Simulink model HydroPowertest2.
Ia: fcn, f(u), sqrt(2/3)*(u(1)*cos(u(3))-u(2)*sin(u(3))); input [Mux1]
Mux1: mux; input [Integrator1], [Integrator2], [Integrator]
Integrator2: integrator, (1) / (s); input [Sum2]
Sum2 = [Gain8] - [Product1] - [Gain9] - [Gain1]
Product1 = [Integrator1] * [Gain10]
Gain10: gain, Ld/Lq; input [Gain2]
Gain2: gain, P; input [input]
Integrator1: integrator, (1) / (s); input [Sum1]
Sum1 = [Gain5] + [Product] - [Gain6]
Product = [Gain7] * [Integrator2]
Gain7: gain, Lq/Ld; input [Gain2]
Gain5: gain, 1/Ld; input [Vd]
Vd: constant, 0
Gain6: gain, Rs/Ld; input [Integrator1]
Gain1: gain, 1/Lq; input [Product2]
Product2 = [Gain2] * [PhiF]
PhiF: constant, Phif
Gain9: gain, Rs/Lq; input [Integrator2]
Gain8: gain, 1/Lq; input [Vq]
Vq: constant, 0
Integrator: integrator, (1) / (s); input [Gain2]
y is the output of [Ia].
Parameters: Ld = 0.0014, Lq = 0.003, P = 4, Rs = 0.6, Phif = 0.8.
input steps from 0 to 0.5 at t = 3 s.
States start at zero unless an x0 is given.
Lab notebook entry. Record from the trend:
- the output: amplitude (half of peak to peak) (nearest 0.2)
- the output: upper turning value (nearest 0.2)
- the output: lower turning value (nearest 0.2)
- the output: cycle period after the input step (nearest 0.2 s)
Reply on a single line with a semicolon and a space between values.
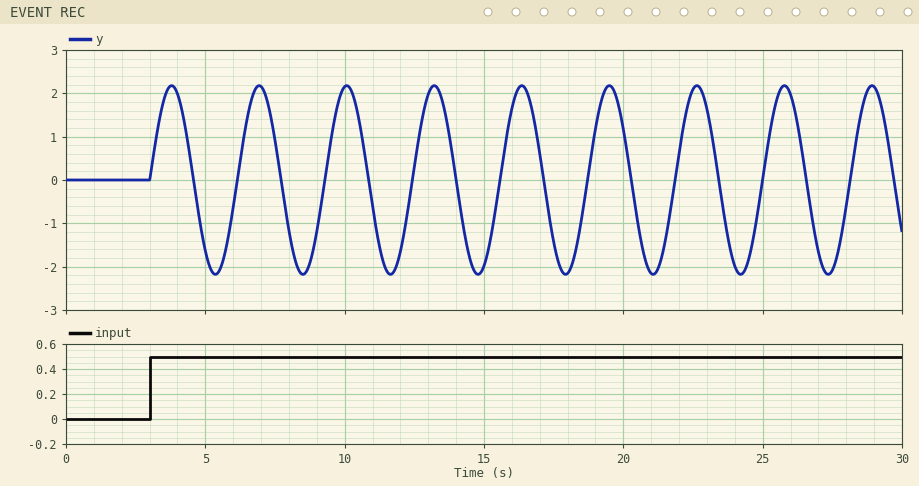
2.2; 2.2; -2.2; 3.2 s
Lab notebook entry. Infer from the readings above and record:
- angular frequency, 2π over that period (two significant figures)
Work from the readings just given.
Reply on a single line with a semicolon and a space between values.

2.0 rad/s
